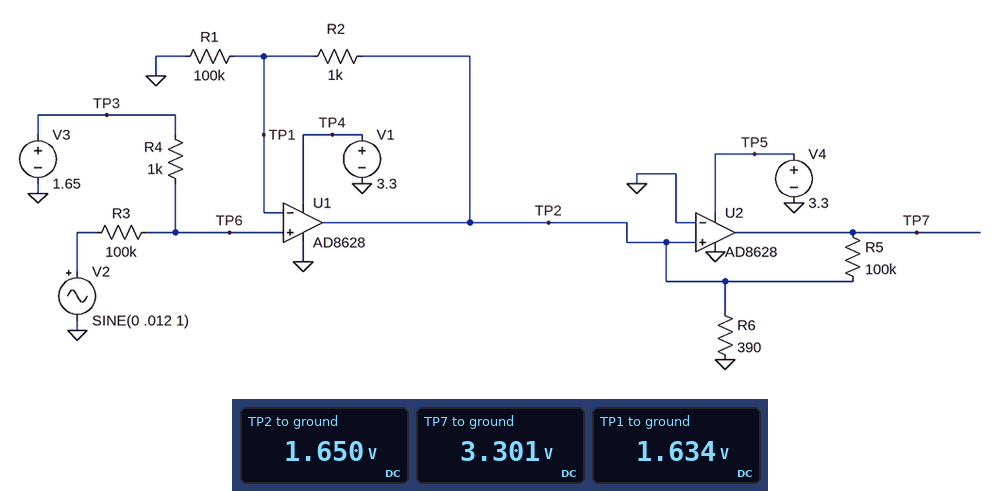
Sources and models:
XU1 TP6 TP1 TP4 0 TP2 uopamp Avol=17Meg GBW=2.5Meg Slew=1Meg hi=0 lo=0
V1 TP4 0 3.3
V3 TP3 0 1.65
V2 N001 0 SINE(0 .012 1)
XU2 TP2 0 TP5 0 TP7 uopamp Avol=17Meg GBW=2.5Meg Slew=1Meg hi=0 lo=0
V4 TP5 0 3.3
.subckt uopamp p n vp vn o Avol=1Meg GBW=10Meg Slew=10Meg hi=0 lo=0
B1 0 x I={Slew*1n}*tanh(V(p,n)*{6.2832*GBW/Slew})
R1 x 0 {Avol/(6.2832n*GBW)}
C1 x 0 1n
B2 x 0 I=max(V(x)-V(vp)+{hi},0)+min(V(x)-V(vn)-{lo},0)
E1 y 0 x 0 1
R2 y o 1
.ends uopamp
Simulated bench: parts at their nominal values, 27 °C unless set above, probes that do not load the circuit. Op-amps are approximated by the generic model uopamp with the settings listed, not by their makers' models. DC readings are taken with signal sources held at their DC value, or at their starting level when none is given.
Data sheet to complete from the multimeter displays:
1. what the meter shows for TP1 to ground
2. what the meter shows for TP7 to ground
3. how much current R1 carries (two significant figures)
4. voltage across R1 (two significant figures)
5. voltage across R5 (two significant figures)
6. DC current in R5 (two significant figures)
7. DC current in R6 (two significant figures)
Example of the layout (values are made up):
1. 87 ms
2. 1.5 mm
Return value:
1. 1.634 V
2. 3.301 V
3. 16 µA
4. 1.6 V
5. 1.7 V
6. 17 µA
7. 4.2 mA
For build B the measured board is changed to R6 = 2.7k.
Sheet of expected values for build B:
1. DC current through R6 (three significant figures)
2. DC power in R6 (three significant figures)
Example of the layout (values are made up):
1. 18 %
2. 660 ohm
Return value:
1. 611 µA
2. 1.01 mW
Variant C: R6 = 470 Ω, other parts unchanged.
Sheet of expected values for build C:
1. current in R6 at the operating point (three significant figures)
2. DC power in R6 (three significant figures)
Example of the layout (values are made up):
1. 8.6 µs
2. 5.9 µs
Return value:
1. 3.51 mA
2. 5.79 mW
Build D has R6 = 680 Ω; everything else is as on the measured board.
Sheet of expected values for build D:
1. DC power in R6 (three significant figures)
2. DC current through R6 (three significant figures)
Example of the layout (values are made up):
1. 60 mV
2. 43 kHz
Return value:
1. 4.00 mW
2. 2.43 mA
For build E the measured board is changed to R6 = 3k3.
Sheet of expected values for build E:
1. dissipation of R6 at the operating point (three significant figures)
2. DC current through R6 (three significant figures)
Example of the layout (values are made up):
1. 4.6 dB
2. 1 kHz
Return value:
1. 825 µW
2. 500 µA
